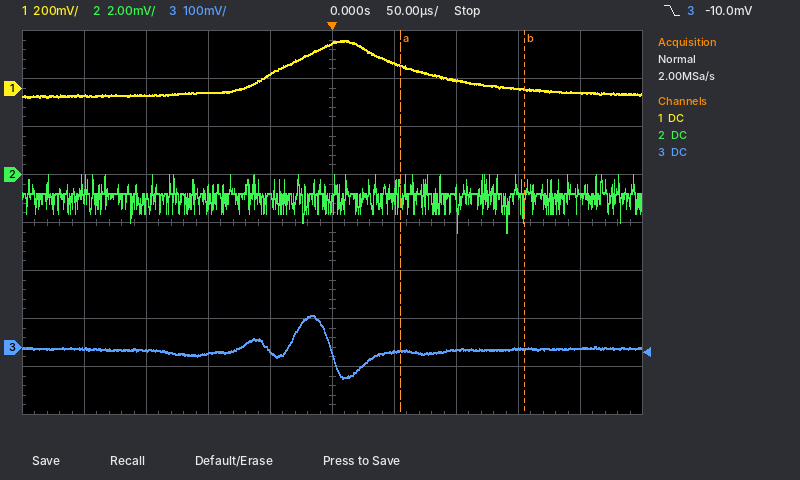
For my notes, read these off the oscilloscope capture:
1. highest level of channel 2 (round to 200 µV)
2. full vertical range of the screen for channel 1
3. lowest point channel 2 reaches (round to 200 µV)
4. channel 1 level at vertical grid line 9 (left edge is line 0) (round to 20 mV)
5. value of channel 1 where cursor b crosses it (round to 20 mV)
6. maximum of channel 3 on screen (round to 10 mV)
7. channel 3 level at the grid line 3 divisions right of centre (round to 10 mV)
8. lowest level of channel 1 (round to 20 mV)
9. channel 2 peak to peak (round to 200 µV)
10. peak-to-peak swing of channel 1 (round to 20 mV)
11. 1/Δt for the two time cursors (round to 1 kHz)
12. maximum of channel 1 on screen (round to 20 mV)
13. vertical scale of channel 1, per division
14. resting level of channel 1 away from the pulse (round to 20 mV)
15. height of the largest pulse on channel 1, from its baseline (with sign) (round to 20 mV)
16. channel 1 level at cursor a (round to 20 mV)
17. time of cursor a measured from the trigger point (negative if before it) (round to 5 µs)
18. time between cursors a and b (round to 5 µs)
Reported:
0.0 mV
1.6 V
-2.4 mV
-20 mV
0 mV
70 mV
0 mV
-40 mV
2.4 mV
240 mV
10 kHz
200 mV
200 mV
-20 mV
+220 mV
100 mV
+55 µs
100 µs
